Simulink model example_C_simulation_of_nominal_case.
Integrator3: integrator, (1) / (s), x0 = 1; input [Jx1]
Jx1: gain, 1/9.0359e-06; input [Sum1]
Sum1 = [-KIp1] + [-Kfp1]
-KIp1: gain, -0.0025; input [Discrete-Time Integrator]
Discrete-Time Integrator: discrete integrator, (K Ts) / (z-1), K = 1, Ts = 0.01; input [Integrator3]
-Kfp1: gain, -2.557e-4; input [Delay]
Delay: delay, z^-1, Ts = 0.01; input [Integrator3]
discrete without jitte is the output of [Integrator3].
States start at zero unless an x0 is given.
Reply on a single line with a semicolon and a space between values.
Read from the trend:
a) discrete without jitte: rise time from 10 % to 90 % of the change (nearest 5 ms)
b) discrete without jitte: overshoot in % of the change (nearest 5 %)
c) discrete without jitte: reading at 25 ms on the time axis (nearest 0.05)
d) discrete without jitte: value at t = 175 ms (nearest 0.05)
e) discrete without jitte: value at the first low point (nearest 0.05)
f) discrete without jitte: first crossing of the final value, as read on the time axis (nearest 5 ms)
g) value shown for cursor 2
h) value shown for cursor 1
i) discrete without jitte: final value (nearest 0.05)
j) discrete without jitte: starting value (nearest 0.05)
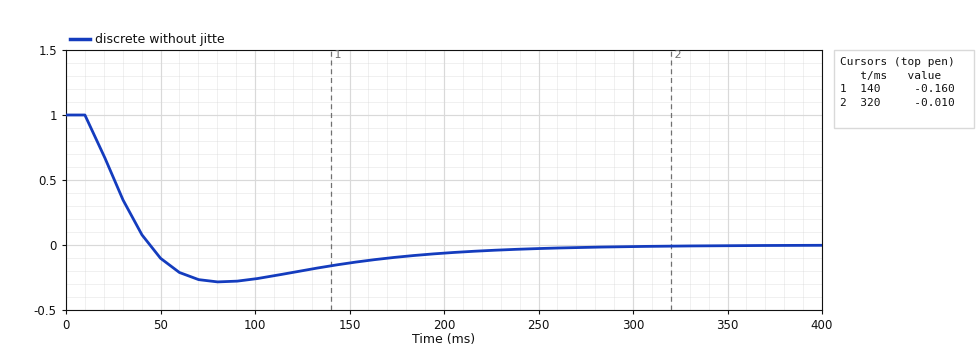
25 ms; 30 %; 0.50; -0.10; -0.30; 45 ms; -0.010; -0.160; 0.00; 1.00
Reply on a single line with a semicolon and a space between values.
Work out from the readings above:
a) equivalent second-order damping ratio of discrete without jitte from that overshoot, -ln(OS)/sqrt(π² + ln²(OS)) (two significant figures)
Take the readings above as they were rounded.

0.36
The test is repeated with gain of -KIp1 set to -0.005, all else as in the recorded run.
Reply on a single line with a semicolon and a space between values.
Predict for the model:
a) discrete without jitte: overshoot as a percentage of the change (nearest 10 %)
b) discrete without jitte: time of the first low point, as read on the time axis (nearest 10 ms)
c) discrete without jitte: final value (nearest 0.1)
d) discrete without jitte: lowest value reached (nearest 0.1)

50 %; 70 ms; 0.0; -0.5
